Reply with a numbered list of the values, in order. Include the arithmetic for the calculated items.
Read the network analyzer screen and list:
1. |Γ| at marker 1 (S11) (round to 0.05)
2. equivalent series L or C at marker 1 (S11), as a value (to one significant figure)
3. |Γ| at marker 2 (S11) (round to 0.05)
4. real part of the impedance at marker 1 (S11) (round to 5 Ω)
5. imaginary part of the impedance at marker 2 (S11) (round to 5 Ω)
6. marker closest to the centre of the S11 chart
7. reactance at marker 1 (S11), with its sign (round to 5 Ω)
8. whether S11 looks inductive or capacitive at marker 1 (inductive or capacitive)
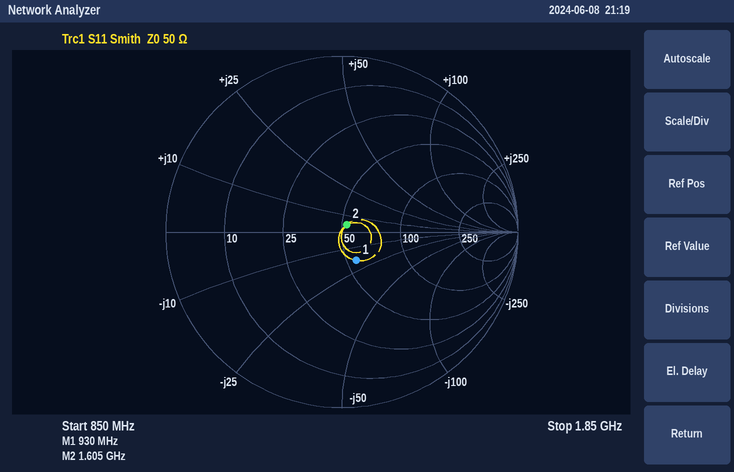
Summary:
1. 0.20
2. C = 1/(2π × 930 MHz × 20 Ω) ≈ 9 pF
3. 0.05
4. 55 Ω
5. +5 Ω
6. marker 2
7. -20 Ω
8. capacitive
